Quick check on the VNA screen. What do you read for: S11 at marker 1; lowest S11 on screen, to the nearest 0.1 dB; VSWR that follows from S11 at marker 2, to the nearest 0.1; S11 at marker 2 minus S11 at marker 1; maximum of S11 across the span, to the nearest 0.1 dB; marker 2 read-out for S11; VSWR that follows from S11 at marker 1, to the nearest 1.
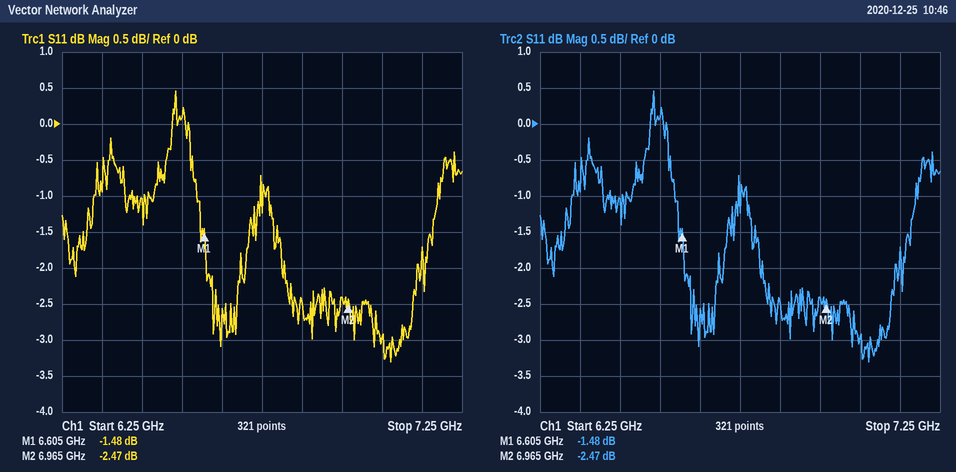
-1.48 dB
-3.3 dB
7.1
-0.99 dB
0.5 dB
-2.47 dB
12
